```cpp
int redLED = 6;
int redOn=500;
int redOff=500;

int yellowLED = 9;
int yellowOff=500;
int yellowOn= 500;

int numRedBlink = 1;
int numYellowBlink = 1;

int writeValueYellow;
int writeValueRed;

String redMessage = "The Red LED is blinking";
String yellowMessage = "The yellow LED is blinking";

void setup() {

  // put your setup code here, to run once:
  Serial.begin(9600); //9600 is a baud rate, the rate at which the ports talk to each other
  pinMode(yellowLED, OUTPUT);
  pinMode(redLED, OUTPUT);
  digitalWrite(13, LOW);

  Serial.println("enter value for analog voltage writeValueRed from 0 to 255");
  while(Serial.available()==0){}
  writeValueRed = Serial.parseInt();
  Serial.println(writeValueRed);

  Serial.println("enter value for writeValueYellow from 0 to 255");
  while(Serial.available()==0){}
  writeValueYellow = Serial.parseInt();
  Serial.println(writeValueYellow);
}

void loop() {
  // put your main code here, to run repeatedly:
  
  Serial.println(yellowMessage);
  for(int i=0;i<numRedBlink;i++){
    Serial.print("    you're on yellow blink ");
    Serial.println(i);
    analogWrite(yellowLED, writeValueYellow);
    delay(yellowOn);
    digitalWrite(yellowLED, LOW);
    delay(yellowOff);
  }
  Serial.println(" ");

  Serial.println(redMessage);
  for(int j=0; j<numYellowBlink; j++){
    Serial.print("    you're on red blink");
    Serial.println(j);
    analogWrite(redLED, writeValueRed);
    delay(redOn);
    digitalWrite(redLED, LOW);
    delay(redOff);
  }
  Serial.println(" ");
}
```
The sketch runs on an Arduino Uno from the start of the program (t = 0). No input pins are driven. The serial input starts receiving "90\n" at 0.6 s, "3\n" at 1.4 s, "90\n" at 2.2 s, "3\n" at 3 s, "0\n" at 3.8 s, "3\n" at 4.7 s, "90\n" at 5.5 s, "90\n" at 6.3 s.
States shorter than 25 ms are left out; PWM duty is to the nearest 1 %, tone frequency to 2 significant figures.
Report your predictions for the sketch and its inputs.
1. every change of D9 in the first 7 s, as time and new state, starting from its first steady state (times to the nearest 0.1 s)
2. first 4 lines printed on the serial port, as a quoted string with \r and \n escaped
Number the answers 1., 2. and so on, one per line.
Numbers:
1. 0 s low; 1.4 s PWM 1 %; 1.9 s low; 3.4 s PWM 1 %; 3.9 s low; 5.4 s PWM 1 %; 5.9 s low
2. "enter value for analog voltage writeValueRed from 0 to 255\r\n90\r\nenter value for writeValueYellow from 0 to 255\r\n3\r\n"
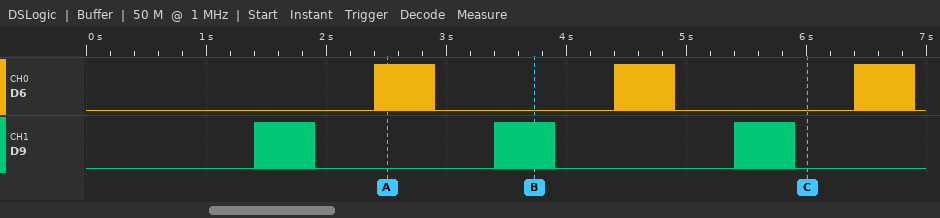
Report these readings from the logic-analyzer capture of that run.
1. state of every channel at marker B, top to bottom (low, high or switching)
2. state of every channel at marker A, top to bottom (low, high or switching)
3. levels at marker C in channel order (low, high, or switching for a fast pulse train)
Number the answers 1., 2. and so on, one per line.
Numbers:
1. D6 low, D9 switching
2. D6 switching, D9 low
3. D6 low, D9 low
